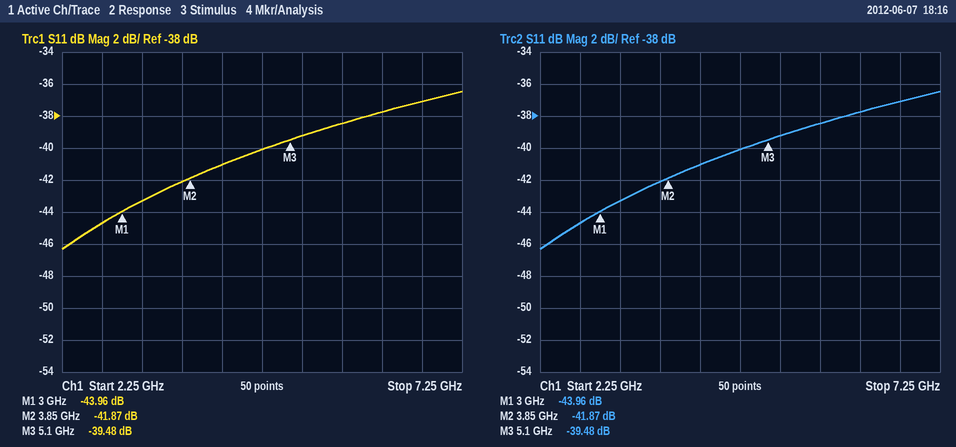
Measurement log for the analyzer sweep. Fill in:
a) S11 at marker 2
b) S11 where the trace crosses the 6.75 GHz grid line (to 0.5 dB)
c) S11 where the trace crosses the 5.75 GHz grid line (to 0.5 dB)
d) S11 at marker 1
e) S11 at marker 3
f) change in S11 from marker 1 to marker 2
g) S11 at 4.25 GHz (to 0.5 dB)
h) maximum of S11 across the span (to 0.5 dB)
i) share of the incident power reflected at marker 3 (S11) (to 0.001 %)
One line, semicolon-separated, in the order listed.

-41.87 dB; -37.0 dB; -38.5 dB; -43.96 dB; -39.48 dB; 2.09 dB; -41.0 dB; -36.5 dB; 0.011 %
